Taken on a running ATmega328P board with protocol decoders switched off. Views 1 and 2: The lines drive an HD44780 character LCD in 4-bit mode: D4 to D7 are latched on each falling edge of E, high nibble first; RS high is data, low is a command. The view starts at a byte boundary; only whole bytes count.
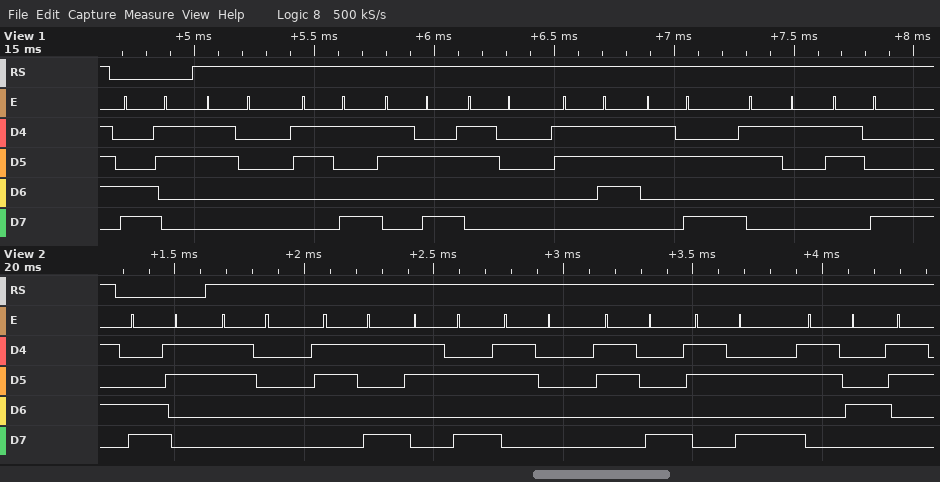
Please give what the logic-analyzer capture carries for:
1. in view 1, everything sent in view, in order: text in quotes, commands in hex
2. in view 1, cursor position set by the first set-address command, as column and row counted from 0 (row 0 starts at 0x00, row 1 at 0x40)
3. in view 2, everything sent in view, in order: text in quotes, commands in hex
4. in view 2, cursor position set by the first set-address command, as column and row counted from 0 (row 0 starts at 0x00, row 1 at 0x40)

0xC3 "09:07:18"
column 3, row 1
0xC3 "09:08:4"
column 3, row 1
